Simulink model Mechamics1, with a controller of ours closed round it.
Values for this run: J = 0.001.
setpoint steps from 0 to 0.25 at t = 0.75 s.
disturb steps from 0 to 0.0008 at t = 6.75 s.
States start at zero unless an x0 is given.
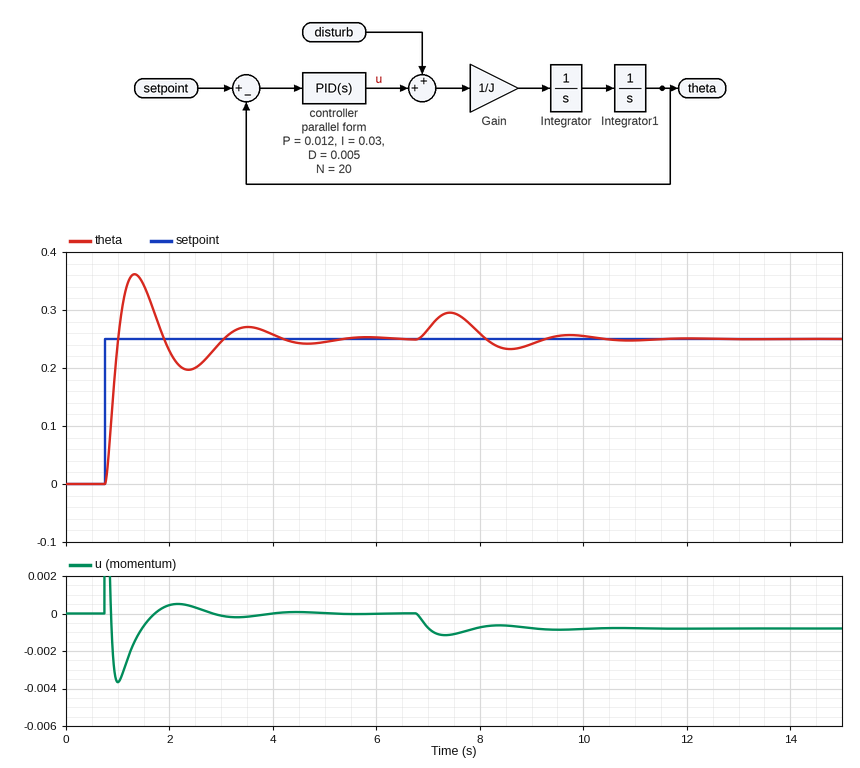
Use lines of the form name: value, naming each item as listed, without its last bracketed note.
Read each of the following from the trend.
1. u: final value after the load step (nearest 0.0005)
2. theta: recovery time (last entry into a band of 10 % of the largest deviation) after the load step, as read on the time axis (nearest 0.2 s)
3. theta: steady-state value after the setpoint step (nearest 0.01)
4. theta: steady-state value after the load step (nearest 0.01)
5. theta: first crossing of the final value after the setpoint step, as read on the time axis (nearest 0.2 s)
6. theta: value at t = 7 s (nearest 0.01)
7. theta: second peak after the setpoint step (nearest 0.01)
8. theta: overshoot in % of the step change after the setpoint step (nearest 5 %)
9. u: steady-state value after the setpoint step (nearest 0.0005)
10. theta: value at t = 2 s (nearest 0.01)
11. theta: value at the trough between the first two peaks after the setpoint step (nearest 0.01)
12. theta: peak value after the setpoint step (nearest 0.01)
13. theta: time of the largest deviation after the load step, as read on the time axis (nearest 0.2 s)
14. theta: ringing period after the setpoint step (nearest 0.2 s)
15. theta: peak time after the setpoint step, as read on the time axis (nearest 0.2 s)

u: final value after the load step: -0.0010
theta: recovery time (last entry into a band of 10 % of the largest deviation) after the load step, as read on the time axis: 10.0 s
theta: steady-state value after the setpoint step: 0.25
theta: steady-state value after the load step: 0.25
theta: first crossing of the final value after the setpoint step, as read on the time axis: 1.0 s
theta: value at t = 7 s: 0.27
theta: second peak after the setpoint step: 0.27
theta: overshoot in % of the step change after the setpoint step: 45 %
u: steady-state value after the setpoint step: 0.0000
theta: value at t = 2 s: 0.23
theta: value at the trough between the first two peaks after the setpoint step: 0.20
theta: peak value after the setpoint step: 0.36
theta: time of the largest deviation after the load step, as read on the time axis: 7.4 s
theta: ringing period after the setpoint step: 2.2 s
theta: peak time after the setpoint step, as read on the time axis: 1.4 s
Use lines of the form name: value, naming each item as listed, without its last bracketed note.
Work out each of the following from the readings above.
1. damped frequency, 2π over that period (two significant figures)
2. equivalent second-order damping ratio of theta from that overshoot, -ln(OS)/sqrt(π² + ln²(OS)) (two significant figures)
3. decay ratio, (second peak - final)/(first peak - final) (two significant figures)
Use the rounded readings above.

damped frequency, 2π over that period: 2.9 rad/s
equivalent second-order damping ratio of theta from that overshoot, -ln(OS)/sqrt(π² + ln²(OS)): 0.25
decay ratio, (second peak - final)/(first peak - final): 0.18
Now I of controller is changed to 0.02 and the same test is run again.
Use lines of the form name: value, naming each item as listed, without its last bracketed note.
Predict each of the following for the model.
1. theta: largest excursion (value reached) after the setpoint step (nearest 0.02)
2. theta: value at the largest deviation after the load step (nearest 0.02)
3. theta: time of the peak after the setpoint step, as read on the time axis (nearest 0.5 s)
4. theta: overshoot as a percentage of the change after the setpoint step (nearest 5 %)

theta: largest excursion (value reached) after the setpoint step: 0.34
theta: value at the largest deviation after the load step: 0.30
theta: time of the peak after the setpoint step, as read on the time axis: 1.5 s
theta: overshoot as a percentage of the change after the setpoint step: 40 %
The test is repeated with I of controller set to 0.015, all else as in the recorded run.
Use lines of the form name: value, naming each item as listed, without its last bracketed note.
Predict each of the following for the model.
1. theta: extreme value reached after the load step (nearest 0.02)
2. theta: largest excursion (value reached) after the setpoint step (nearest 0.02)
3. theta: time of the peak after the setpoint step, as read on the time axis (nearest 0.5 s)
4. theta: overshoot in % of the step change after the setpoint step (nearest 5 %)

theta: extreme value reached after the load step: 0.30
theta: largest excursion (value reached) after the setpoint step: 0.34
theta: time of the peak after the setpoint step, as read on the time axis: 1.5 s
theta: overshoot in % of the step change after the setpoint step: 35 %
